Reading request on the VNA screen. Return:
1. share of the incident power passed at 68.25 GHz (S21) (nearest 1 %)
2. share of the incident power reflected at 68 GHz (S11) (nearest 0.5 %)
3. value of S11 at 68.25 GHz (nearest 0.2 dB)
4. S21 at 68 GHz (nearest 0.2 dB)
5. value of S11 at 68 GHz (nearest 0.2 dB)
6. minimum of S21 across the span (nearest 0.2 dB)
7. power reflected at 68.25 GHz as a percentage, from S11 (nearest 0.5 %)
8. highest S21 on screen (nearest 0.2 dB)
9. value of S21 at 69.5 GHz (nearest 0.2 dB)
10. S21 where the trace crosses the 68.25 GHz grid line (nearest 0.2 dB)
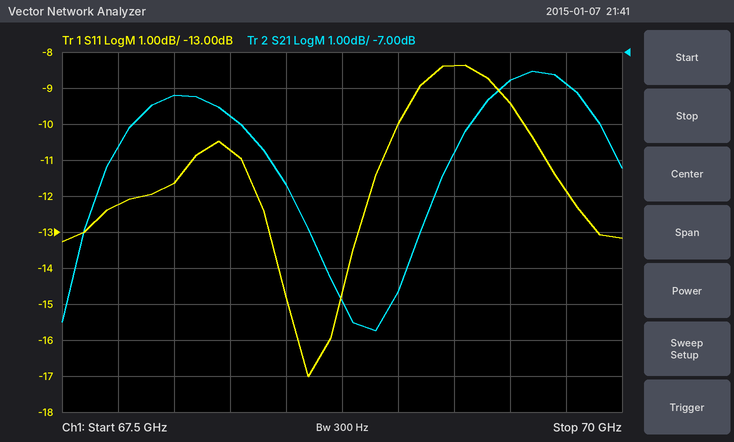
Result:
13 %
7.0 %
-10.8 dB
-8.2 dB
-11.6 dB
-14.8 dB
8.5 %
-7.6 dB
-7.8 dB
-8.8 dB
